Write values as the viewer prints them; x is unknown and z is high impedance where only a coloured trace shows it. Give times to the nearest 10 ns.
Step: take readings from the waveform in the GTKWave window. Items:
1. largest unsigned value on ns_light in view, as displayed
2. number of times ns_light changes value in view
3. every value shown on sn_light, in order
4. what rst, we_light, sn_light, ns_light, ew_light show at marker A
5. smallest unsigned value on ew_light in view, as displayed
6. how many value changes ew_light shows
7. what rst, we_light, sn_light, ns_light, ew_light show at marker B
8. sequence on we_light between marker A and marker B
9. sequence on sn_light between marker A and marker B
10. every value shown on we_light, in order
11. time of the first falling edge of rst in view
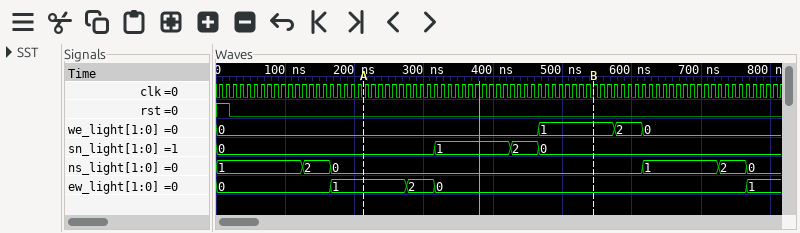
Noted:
2
5
0, 1, 2, 0
rst=0, we_light=0, sn_light=0, ns_light=0, ew_light=1
0
4
rst=0, we_light=1, sn_light=0, ns_light=0, ew_light=0
0, 1
0, 1, 2, 0
0, 1, 2, 0
20 ns
